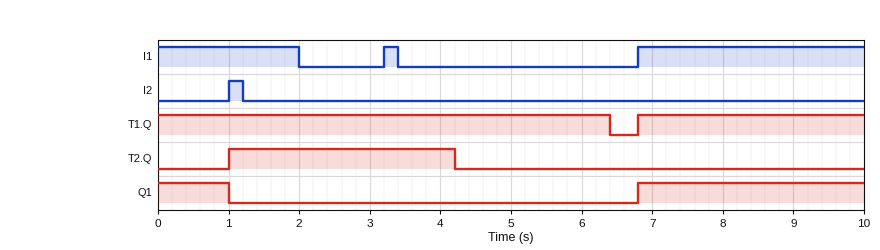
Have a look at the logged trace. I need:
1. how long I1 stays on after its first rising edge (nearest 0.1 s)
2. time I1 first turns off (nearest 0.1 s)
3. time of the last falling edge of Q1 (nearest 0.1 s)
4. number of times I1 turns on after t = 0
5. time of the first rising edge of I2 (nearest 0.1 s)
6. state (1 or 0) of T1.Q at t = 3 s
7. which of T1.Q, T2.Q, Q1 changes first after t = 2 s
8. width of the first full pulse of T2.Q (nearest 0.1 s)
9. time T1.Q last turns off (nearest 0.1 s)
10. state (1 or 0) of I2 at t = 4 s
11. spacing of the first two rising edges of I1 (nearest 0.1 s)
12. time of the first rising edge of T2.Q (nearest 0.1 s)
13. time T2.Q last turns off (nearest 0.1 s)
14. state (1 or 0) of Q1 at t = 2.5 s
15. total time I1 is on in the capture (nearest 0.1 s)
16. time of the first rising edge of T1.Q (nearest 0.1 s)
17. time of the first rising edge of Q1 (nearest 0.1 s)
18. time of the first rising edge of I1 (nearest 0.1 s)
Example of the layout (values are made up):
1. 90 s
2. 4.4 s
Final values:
1. 0.2 s
2. 2.0 s
3. 1.0 s
4. 2
5. 1.0 s
6. 1
7. T2.Q
8. 3.2 s
9. 6.4 s
10. 0
11. 3.6 s
12. 1.0 s
13. 4.2 s
14. 0
15. 5.4 s
16. 6.8 s
17. 6.8 s
18. 3.2 s
